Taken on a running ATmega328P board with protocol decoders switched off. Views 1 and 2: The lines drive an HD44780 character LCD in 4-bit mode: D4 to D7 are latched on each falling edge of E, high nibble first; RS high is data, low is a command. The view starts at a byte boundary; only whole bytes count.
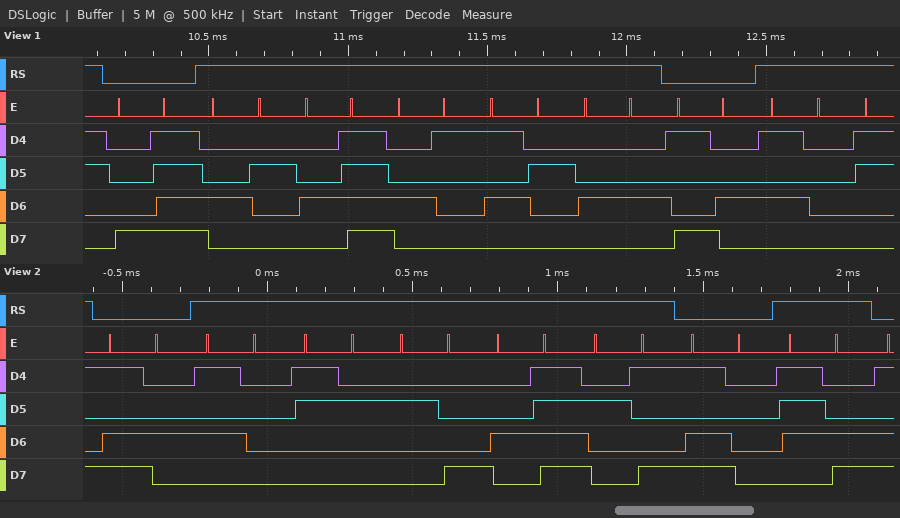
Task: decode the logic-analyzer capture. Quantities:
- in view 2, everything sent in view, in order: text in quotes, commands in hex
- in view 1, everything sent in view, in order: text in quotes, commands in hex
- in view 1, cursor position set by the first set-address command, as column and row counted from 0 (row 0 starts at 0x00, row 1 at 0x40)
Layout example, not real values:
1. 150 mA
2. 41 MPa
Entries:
1. 0xD4 "P2(O)" 0xD0 "|"
2. 0x8F "BOARD" 0x94 "P"
3. column 15, row 0
